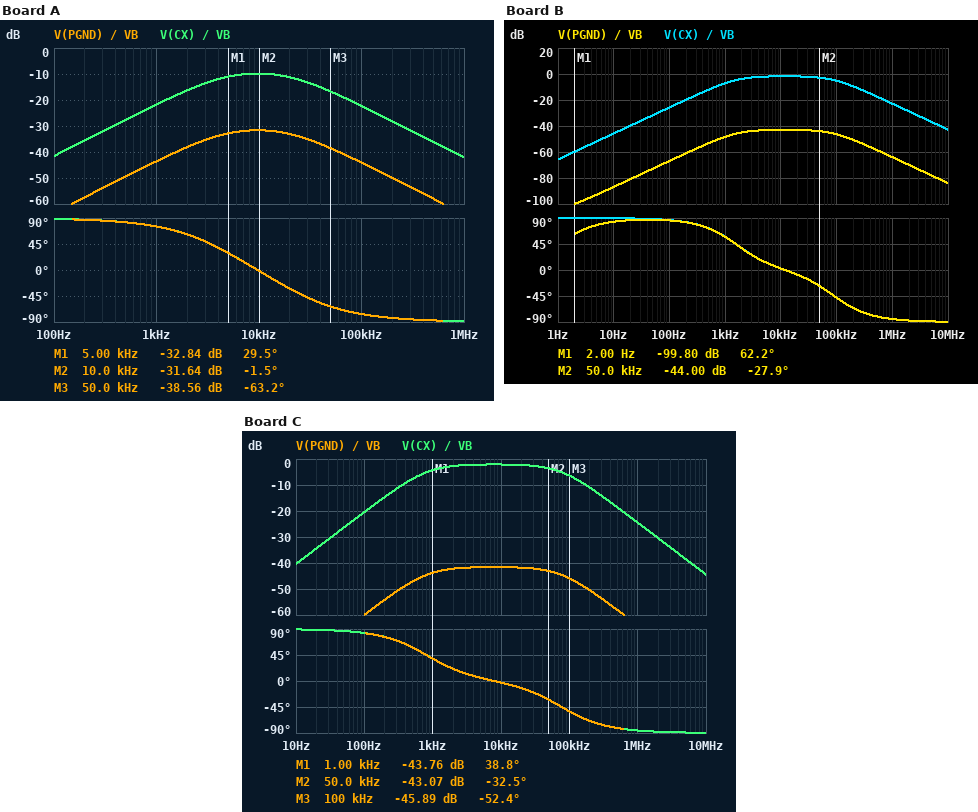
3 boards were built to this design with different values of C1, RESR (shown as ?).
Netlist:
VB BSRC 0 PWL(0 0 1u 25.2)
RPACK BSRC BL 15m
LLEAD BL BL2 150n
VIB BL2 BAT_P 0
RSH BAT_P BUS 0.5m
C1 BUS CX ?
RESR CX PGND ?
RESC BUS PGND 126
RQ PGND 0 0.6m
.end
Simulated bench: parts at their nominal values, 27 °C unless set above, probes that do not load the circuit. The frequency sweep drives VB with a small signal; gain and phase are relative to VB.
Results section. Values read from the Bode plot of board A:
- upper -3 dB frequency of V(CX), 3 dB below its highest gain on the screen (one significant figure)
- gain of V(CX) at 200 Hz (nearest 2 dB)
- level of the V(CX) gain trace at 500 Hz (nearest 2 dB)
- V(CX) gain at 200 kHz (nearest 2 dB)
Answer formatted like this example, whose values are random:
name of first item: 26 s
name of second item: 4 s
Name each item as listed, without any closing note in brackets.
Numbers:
upper -3 dB frequency of V(CX), 3 dB below its highest gain on the screen: 30 kHz
gain of V(CX) at 200 Hz: -36 dB
level of the V(CX) gain trace at 500 Hz: -28 dB
V(CX) gain at 200 kHz: -28 dB
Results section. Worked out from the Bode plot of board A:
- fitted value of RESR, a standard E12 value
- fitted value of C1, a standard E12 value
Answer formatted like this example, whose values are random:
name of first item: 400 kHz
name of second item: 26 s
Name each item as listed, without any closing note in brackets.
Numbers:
fitted value of RESR, a standard E12 value: 6.8 mΩ
fitted value of C1, a standard E12 value: 1.8 mF
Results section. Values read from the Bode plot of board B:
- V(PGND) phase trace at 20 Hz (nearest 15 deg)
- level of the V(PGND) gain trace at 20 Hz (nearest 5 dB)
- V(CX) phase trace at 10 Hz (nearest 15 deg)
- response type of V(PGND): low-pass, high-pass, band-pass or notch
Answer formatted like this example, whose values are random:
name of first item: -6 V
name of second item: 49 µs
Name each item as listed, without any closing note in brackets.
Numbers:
V(PGND) phase trace at 20 Hz: 90 deg
level of the V(PGND) gain trace at 20 Hz: -80 dB
V(CX) phase trace at 10 Hz: 90 deg
response type of V(PGND): low-pass, high-pass, band-pass or notch: band-pass
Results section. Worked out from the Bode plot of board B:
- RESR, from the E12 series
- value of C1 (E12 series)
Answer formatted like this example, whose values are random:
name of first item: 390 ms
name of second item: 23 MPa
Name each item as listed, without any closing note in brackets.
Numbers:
RESR, from the E12 series: 0.068 Ω
value of C1: 1.2 mF
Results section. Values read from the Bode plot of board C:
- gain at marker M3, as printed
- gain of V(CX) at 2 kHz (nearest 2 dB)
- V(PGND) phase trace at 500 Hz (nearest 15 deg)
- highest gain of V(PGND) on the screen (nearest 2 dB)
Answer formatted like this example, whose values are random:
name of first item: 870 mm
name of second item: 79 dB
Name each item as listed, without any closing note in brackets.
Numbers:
gain at marker M3, as printed: -45.89 dB
gain of V(CX) at 2 kHz: -2 dB
V(PGND) phase trace at 500 Hz: 60 deg
highest gain of V(PGND) on the screen: -42 dB
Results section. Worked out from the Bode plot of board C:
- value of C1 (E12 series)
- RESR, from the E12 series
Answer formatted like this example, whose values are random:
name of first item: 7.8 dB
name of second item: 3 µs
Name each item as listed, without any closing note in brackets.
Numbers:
value of C1: 2.7 mF
RESR, from the E12 series: 0.056 Ω
